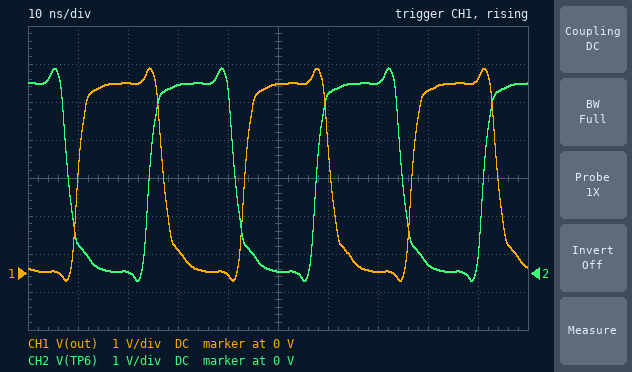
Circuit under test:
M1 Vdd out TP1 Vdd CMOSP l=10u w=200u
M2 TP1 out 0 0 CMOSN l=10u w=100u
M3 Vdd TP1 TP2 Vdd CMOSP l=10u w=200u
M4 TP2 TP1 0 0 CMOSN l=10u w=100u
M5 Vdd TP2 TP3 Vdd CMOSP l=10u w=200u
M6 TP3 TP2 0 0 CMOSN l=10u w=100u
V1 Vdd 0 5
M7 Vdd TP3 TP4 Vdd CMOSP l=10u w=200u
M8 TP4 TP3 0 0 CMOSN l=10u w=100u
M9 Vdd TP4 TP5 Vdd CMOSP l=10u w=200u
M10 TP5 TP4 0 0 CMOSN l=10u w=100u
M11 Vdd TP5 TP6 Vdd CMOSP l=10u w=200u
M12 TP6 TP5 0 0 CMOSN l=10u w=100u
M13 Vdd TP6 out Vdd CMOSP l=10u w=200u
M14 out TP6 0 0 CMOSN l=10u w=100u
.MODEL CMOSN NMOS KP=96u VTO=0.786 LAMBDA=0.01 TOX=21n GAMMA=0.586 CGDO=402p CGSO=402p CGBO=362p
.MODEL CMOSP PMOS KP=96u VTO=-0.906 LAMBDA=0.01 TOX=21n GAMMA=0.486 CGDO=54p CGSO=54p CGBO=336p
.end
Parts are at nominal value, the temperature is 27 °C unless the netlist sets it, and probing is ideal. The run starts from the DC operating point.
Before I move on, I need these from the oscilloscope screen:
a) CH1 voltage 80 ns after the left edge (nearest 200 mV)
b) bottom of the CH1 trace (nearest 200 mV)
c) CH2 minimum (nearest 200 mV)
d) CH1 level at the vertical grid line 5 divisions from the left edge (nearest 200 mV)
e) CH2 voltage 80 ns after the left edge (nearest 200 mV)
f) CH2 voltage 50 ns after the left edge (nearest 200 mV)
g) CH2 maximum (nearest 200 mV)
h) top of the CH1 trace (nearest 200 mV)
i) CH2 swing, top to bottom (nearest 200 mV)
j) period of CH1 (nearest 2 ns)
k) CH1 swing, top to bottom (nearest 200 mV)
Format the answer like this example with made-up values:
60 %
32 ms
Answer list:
4.8 V
-200 mV
-200 mV
5.0 V
200 mV
0 V
5.4 V
5.4 V
5.6 V
34 ns
5.6 V
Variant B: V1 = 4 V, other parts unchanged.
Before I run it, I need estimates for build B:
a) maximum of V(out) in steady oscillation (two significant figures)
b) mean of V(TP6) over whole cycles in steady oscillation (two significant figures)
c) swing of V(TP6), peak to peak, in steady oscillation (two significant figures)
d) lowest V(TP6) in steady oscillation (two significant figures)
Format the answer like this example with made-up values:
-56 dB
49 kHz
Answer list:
4.3 V
2.1 V
4.5 V
-180 mV
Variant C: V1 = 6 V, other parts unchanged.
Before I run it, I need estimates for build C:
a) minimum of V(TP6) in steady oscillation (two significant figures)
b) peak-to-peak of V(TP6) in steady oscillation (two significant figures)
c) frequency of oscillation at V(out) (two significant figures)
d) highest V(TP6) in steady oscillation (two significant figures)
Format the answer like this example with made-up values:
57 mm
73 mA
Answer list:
-230 mV
6.7 V
39 MHz
6.4 V
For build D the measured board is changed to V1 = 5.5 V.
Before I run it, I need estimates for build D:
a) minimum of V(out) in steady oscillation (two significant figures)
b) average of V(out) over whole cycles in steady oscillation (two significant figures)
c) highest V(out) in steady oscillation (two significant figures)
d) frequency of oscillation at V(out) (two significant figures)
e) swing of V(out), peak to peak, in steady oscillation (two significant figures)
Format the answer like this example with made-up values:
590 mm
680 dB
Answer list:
-220 mV
2.9 V
5.9 V
34 MHz
6.1 V
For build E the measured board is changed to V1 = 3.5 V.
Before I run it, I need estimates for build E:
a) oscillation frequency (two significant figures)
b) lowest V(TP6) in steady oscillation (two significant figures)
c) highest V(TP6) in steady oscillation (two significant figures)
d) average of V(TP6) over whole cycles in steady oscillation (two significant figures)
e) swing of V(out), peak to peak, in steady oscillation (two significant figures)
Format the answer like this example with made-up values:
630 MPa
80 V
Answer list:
17 MHz
-170 mV
3.8 V
1.8 V
4.0 V
